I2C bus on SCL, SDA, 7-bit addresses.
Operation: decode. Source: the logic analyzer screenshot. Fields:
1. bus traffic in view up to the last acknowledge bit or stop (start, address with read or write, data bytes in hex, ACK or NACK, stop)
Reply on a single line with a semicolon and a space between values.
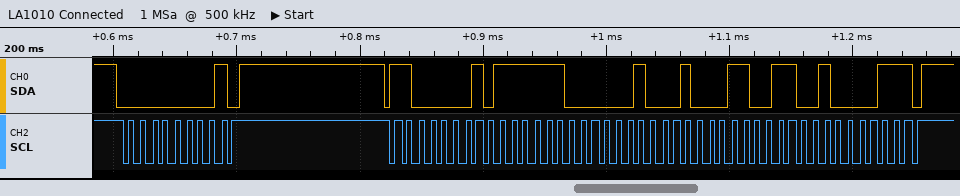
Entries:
start, address 00 write NACK, stop, start, address 60 read ACK, FC ACK, 11 ACK, 33 ACK, 43 NACK, stop
